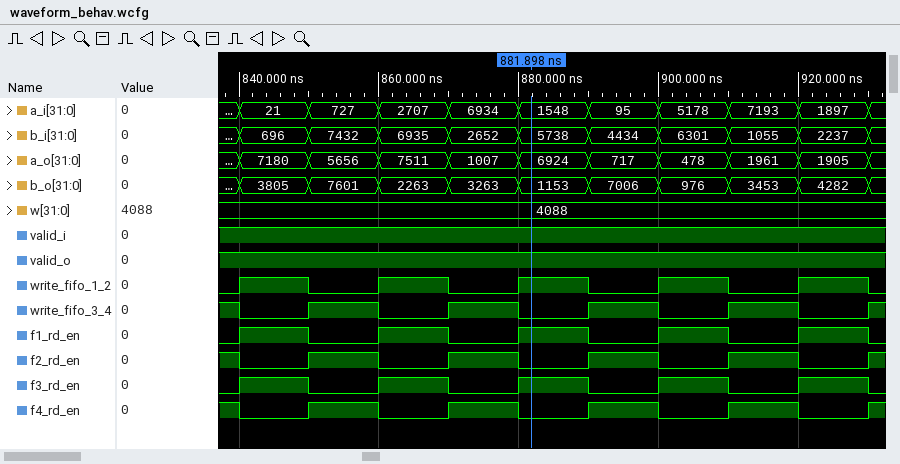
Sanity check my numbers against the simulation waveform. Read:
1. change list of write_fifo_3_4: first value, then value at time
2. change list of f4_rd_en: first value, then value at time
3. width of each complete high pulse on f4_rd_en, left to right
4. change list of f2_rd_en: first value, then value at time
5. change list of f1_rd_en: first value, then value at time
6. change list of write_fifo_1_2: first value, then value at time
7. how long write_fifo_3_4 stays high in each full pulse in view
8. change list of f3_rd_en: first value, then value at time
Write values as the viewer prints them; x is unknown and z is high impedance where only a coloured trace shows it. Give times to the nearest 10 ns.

1, 0 at 840 ns, 1 at 850 ns, 0 at 860 ns, 1 at 870 ns, 0 at 880 ns, 1 at 890 ns, 0 at 900 ns, 1 at 910 ns, 0 at 920 ns, 1 at 930 ns
1, 0 at 840 ns, 1 at 850 ns, 0 at 860 ns, 1 at 870 ns, 0 at 880 ns, 1 at 890 ns, 0 at 900 ns, 1 at 910 ns, 0 at 920 ns, 1 at 930 ns
10 ns, 10 ns, 10 ns, 10 ns
1, 0 at 840 ns, 1 at 850 ns, 0 at 860 ns, 1 at 870 ns, 0 at 880 ns, 1 at 890 ns, 0 at 900 ns, 1 at 910 ns, 0 at 920 ns, 1 at 930 ns
0, 1 at 840 ns, 0 at 850 ns, 1 at 860 ns, 0 at 870 ns, 1 at 880 ns, 0 at 890 ns, 1 at 900 ns, 0 at 910 ns, 1 at 920 ns, 0 at 930 ns
0, 1 at 840 ns, 0 at 850 ns, 1 at 860 ns, 0 at 870 ns, 1 at 880 ns, 0 at 890 ns, 1 at 900 ns, 0 at 910 ns, 1 at 920 ns, 0 at 930 ns
10 ns, 10 ns, 10 ns, 10 ns
0, 1 at 840 ns, 0 at 850 ns, 1 at 860 ns, 0 at 870 ns, 1 at 880 ns, 0 at 890 ns, 1 at 900 ns, 0 at 910 ns, 1 at 920 ns, 0 at 930 ns
